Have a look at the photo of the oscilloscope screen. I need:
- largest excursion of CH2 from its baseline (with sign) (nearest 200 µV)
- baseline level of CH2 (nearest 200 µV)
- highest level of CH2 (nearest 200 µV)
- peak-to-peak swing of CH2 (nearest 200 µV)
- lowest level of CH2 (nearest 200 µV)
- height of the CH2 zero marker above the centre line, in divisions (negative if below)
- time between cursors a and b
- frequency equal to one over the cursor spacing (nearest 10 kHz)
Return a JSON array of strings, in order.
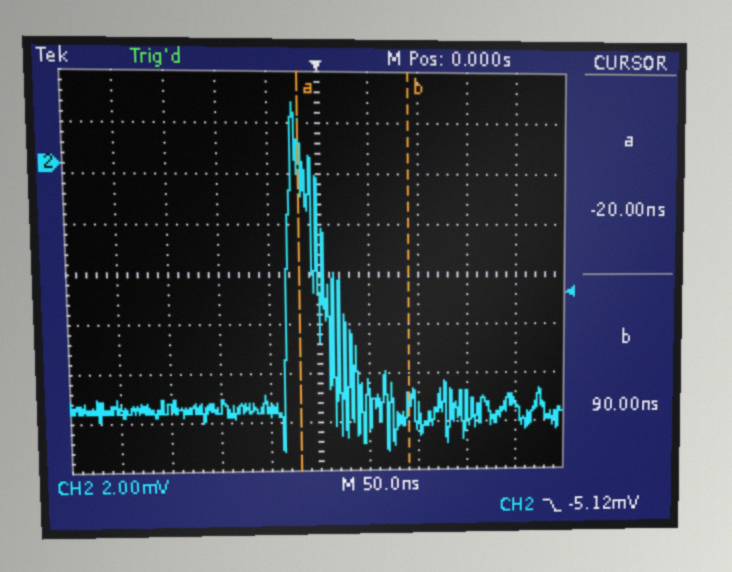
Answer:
["+12.2 mV", "-9.8 mV", "2.4 mV", "14.0 mV", "-11.6 mV", "+2.2 div", "110 ns", "9.09 MHz"]
